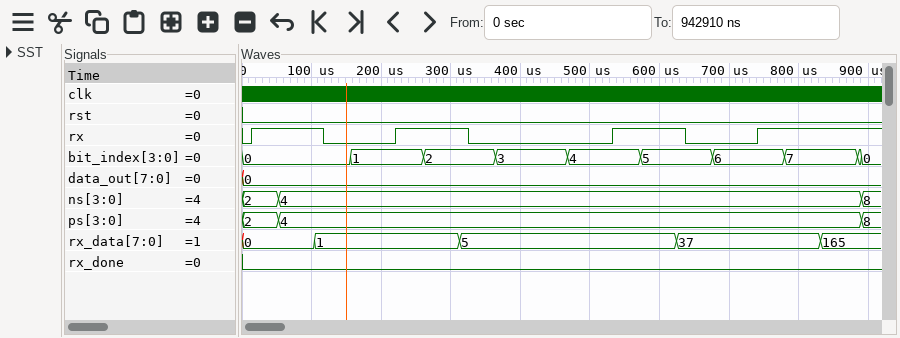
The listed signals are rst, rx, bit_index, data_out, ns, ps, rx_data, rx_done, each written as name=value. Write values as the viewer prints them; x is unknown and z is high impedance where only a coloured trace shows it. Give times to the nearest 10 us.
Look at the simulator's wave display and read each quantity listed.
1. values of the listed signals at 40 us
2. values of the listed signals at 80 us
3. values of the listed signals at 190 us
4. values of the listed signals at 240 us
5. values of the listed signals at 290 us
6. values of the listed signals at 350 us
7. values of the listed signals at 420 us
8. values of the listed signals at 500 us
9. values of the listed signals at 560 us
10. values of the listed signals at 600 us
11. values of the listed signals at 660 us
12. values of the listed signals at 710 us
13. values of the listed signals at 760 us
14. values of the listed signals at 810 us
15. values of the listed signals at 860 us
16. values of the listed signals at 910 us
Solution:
rst=0, rx=1, bit_index=0, data_out=0, ns=2, ps=2, rx_data=0, rx_done=0
rst=0, rx=1, bit_index=0, data_out=0, ns=4, ps=4, rx_data=0, rx_done=0
rst=0, rx=0, bit_index=1, data_out=0, ns=4, ps=4, rx_data=1, rx_done=0
rst=0, rx=1, bit_index=1, data_out=0, ns=4, ps=4, rx_data=1, rx_done=0
rst=0, rx=1, bit_index=2, data_out=0, ns=4, ps=4, rx_data=1, rx_done=0
rst=0, rx=0, bit_index=2, data_out=0, ns=4, ps=4, rx_data=5, rx_done=0
rst=0, rx=0, bit_index=3, data_out=0, ns=4, ps=4, rx_data=5, rx_done=0
rst=0, rx=0, bit_index=4, data_out=0, ns=4, ps=4, rx_data=5, rx_done=0
rst=0, rx=1, bit_index=4, data_out=0, ns=4, ps=4, rx_data=5, rx_done=0
rst=0, rx=1, bit_index=5, data_out=0, ns=4, ps=4, rx_data=5, rx_done=0
rst=0, rx=0, bit_index=5, data_out=0, ns=4, ps=4, rx_data=37, rx_done=0
rst=0, rx=0, bit_index=6, data_out=0, ns=4, ps=4, rx_data=37, rx_done=0
rst=0, rx=1, bit_index=6, data_out=0, ns=4, ps=4, rx_data=37, rx_done=0
rst=0, rx=1, bit_index=7, data_out=0, ns=4, ps=4, rx_data=37, rx_done=0
rst=0, rx=1, bit_index=7, data_out=0, ns=4, ps=4, rx_data=165, rx_done=0
rst=0, rx=1, bit_index=0, data_out=0, ns=8, ps=8, rx_data=165, rx_done=0
